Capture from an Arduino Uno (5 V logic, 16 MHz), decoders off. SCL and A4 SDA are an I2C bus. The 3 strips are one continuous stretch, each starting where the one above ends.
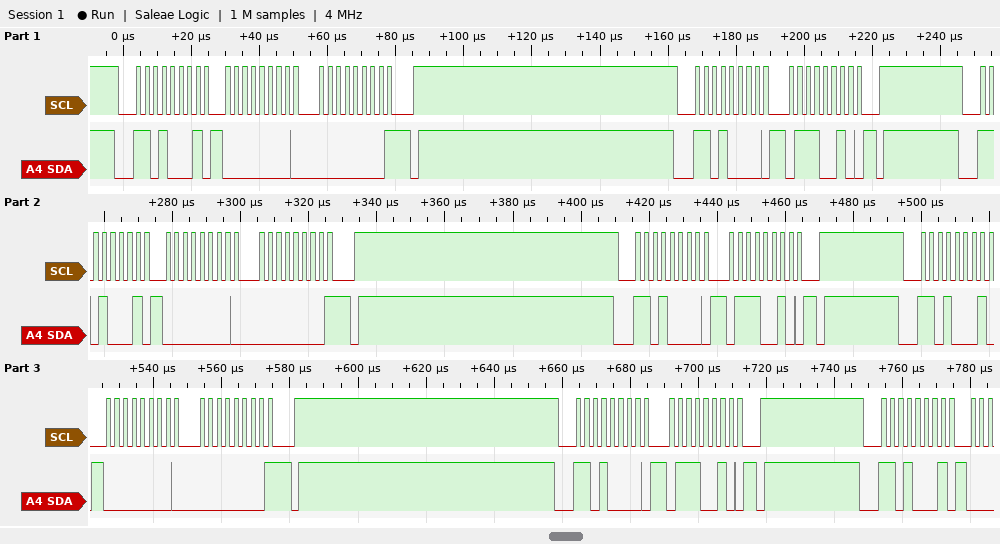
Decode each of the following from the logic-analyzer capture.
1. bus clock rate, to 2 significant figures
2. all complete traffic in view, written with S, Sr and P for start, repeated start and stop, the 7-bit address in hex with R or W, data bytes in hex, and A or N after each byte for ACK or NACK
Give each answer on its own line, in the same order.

400 kHz
S 68R A 00 A 00 N P S 68W A 72 A P S 68R A 00 A 00 N P S 68W A 72 A P S 68R A 00 A 00 N P S 68W A 72 A P S 68R A
